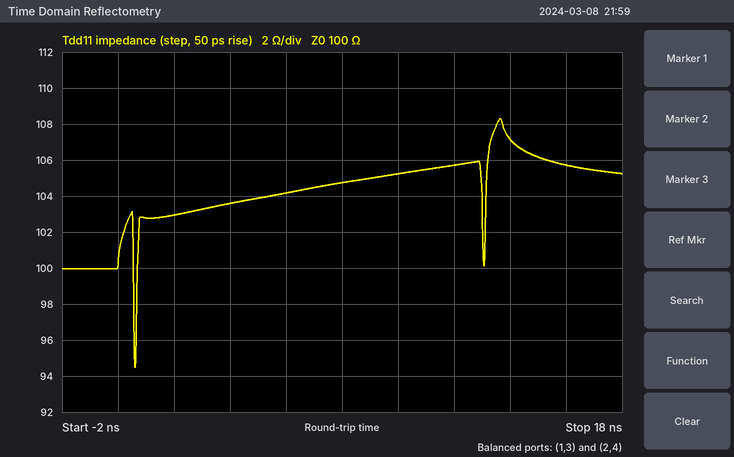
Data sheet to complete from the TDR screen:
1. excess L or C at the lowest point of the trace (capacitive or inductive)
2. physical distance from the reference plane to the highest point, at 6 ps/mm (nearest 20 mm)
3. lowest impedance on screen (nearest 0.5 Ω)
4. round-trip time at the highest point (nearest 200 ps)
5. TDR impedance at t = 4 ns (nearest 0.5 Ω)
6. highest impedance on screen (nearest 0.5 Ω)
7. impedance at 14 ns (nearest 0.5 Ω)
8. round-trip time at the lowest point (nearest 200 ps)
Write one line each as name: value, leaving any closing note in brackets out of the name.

excess L or C at the lowest point of the trace: capacitive
physical distance from the reference plane to the highest point, at 6 ps/mm: 1.14 m
lowest impedance on screen: 94.5 Ω
round-trip time at the highest point: 13.6 ns
TDR impedance at t = 4 ns: 103.5 Ω
highest impedance on screen: 108.5 Ω
impedance at 14 ns: 107.0 Ω
round-trip time at the lowest point: 600 ps
